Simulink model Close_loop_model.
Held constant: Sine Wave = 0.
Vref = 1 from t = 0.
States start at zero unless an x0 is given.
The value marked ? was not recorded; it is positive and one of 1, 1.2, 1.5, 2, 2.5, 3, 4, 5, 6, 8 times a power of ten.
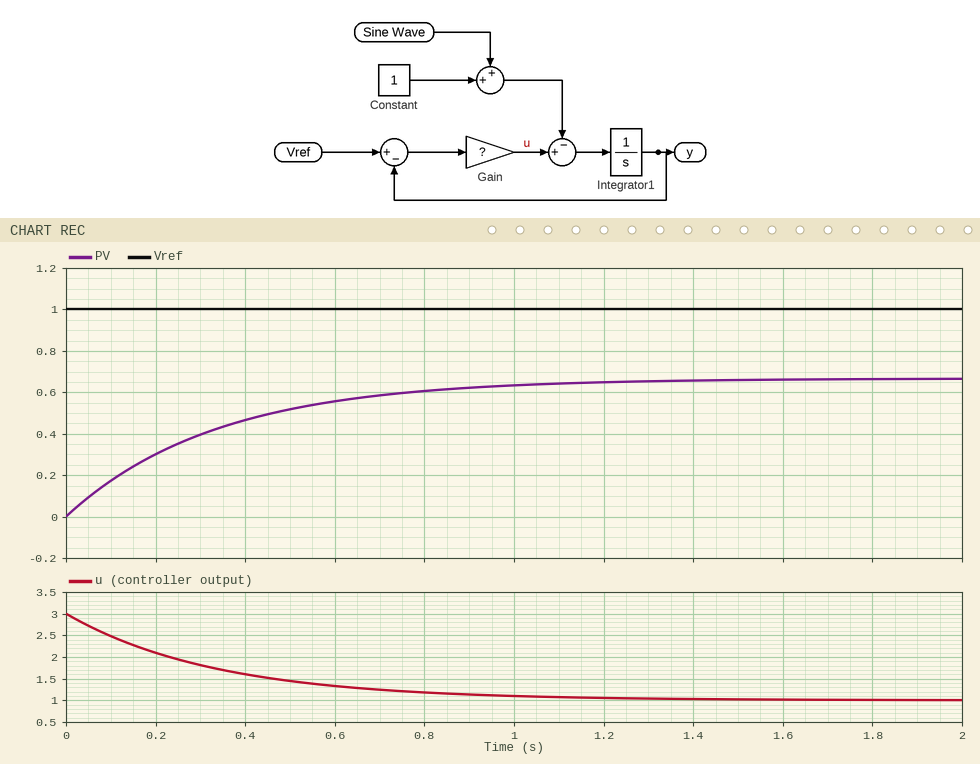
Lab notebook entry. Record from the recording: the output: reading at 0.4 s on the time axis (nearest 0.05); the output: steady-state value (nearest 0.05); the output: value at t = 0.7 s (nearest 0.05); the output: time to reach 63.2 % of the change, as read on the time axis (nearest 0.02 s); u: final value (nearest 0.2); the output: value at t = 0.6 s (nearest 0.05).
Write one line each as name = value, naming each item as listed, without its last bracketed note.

the output: reading at 0.4 s on the time axis = 0.45
the output: steady-state value = 0.65
the output: value at t = 0.7 s = 0.60
the output: time to reach 63.2 % of the change, as read on the time axis = 0.34 s
u: final value = 1.0
the output: value at t = 0.6 s = 0.55
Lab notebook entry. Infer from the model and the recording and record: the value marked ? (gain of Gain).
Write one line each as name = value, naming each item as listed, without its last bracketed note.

the value marked ? = 3
